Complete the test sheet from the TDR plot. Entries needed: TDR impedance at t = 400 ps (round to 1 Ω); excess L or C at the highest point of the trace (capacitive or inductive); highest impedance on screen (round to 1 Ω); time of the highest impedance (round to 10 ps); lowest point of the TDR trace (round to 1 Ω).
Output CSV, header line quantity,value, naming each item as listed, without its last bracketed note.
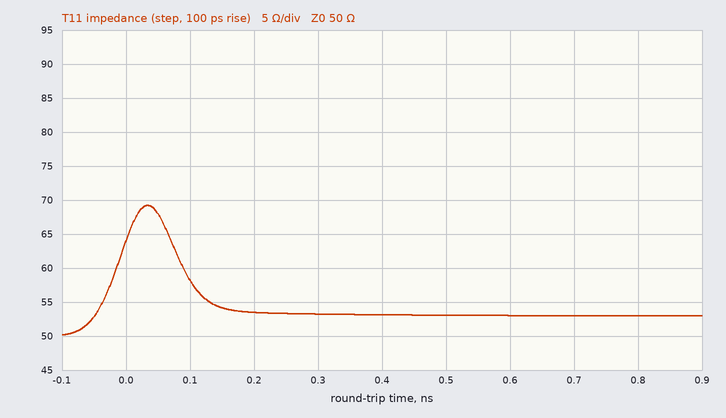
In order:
quantity,value
TDR impedance at t = 400 ps,53 Ω
excess L or C at the highest point of the trace,inductive
highest impedance on screen,69 Ω
time of the highest impedance,30 ps
lowest point of the TDR trace,50 Ω
